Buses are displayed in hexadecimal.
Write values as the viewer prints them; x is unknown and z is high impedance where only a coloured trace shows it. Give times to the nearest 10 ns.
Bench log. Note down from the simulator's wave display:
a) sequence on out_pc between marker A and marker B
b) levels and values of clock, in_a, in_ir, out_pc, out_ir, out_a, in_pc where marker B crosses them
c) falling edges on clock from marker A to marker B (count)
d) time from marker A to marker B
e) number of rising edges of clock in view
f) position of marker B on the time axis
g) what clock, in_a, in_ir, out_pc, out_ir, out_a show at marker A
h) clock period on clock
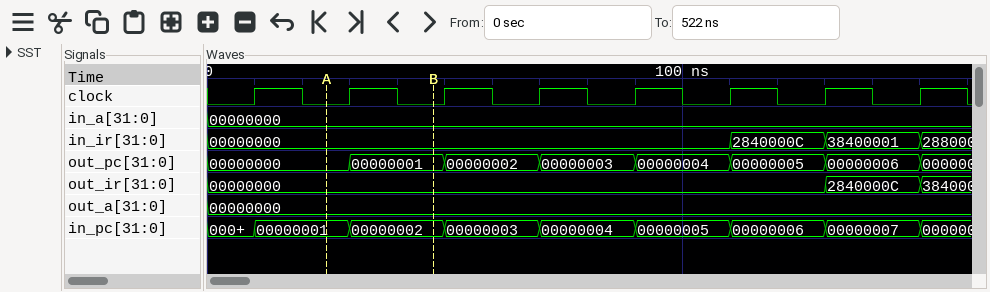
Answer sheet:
00000000, 00000001
clock=0, in_a=00000000, in_ir=00000000, out_pc=00000001, out_ir=00000000, out_a=00000000, in_pc=00000002
1
20 ns
8
50 ns
clock=0, in_a=00000000, in_ir=00000000, out_pc=00000000, out_ir=00000000, out_a=00000000
20 ns
